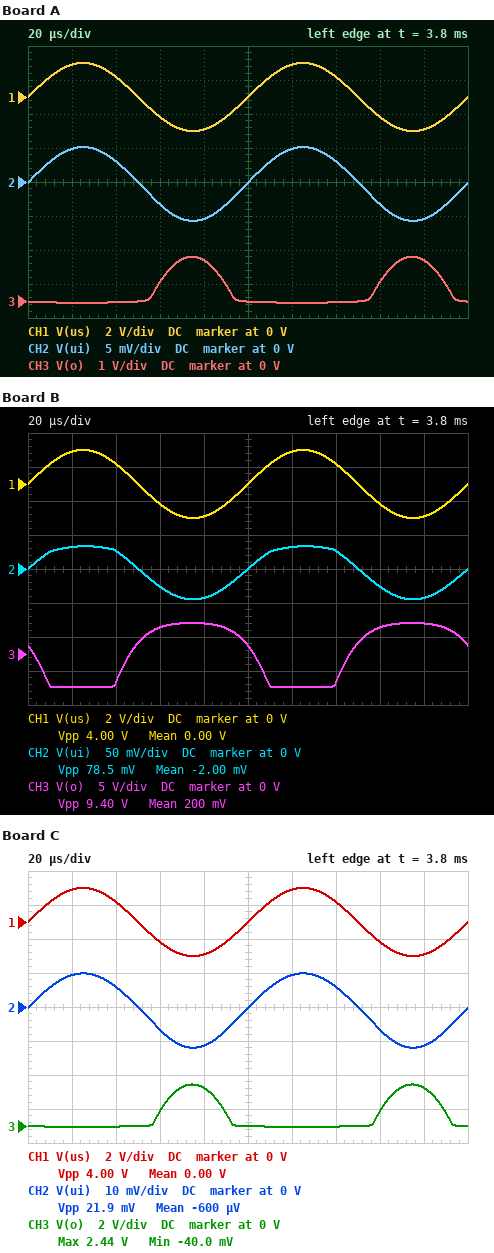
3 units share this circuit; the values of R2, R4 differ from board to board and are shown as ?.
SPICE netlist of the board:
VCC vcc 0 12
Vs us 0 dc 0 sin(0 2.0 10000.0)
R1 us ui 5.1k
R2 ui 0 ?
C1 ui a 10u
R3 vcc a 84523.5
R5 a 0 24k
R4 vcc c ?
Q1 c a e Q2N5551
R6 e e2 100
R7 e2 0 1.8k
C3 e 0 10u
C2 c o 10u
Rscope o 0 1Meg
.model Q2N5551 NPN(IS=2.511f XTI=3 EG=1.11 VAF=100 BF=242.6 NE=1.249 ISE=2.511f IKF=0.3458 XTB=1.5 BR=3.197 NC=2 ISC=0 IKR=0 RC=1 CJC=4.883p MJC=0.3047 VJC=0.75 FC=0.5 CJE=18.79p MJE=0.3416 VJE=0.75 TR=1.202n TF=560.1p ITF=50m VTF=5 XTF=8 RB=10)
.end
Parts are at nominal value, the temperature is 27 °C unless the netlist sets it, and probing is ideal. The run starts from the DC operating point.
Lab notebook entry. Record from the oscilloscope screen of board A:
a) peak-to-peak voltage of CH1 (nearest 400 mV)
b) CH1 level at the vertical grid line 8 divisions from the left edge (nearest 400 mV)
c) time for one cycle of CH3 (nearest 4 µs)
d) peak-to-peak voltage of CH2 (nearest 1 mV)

4.0 V
-1.2 V
100 µs
11 mV
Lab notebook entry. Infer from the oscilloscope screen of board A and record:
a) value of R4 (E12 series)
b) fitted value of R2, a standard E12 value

12 kΩ
15 Ω
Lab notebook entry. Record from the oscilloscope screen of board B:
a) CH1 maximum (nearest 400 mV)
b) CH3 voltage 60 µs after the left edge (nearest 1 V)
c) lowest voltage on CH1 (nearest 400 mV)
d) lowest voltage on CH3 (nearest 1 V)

2.0 V
4 V
-2.0 V
-5 V
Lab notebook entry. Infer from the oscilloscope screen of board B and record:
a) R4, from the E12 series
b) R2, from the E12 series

5.6 kΩ
120 Ω
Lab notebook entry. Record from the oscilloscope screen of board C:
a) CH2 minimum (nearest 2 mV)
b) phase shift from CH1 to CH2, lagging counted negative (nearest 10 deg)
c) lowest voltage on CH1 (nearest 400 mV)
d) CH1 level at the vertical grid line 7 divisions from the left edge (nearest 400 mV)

-12 mV
0 deg
-2.0 V
1.2 V
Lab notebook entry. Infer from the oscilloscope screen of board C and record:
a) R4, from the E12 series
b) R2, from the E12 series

15 kΩ
33 Ω
